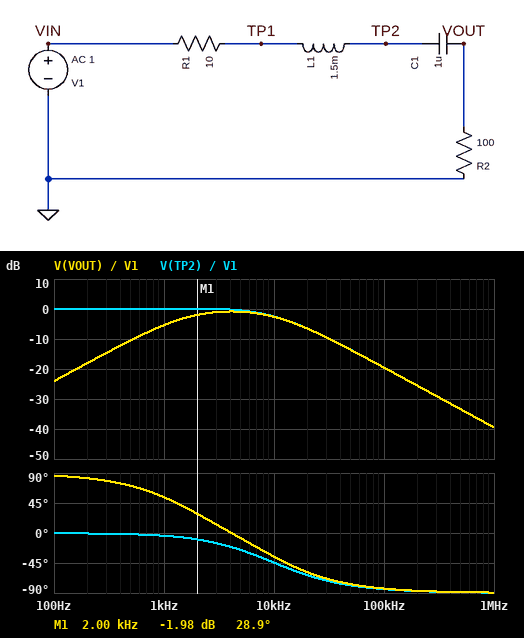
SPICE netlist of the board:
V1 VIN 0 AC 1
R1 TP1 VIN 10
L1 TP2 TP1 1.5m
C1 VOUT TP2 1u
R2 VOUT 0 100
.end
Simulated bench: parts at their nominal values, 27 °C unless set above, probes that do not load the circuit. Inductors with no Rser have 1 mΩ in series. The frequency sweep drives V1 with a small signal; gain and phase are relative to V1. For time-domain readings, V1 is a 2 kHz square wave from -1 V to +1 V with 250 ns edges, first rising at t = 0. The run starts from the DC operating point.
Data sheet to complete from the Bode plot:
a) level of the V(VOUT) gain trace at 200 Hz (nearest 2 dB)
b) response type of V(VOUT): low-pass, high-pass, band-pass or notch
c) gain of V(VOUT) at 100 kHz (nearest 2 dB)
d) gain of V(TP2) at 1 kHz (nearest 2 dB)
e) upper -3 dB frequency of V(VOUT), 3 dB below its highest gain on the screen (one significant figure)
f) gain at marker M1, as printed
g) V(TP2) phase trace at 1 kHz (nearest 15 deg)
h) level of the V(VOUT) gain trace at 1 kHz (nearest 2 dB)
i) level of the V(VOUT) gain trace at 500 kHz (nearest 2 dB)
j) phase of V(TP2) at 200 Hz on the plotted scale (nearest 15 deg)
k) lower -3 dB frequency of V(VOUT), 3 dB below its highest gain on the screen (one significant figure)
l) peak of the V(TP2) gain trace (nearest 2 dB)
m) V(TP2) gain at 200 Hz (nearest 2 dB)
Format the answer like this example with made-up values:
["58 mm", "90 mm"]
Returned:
["-18 dB", "band-pass", "-20 dB", "0 dB", "10 kHz", "-1.98 dB", "0 deg", "-6 dB", "-34 dB", "0 deg", "1 kHz", "0 dB", "0 dB"]
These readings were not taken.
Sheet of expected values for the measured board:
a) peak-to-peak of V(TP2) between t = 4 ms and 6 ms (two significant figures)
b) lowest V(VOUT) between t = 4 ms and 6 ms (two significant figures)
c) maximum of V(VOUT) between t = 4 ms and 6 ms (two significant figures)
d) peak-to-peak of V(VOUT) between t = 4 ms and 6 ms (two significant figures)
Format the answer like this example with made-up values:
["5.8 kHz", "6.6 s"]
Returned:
["2.1 V", "-1.4 V", "1.4 V", "2.7 V"]
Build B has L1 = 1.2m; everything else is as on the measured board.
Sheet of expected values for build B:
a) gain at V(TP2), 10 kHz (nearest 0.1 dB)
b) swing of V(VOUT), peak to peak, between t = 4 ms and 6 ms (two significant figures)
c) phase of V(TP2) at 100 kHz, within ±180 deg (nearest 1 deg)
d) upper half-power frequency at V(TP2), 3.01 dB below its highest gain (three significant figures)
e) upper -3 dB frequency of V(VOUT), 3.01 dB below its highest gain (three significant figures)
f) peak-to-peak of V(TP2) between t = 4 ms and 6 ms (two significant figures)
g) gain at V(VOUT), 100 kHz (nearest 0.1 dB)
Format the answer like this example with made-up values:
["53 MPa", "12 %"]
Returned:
["-1.8 dB", "2.8 V", "-83 deg", "13.4 kHz", "15.9 kHz", "2.0 V", "-17.6 dB"]
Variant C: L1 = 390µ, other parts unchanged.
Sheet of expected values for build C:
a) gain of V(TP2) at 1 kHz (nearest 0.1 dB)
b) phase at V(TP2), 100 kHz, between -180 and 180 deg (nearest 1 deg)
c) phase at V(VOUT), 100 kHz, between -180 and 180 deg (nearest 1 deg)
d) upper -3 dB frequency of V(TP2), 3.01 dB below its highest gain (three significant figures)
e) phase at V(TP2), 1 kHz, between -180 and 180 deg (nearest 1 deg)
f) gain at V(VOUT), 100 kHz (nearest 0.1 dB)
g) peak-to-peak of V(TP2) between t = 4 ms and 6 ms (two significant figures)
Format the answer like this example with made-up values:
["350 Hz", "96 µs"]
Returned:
["-0.2 dB", "-67 deg", "-66 deg", "38.1 kHz", "-3 deg", "-8.5 dB", "2.0 V"]
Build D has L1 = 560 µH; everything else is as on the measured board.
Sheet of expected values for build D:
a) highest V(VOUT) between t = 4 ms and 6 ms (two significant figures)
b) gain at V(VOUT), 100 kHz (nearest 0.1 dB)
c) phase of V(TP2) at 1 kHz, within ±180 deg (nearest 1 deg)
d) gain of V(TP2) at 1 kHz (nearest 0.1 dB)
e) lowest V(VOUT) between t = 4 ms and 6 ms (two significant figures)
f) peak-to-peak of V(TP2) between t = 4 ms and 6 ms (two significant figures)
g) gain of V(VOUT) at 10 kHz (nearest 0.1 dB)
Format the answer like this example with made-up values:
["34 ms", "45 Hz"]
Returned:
["1.5 V", "-11.3 dB", "-3 deg", "-0.1 dB", "-1.5 V", "2.0 V", "-1.0 dB"]
